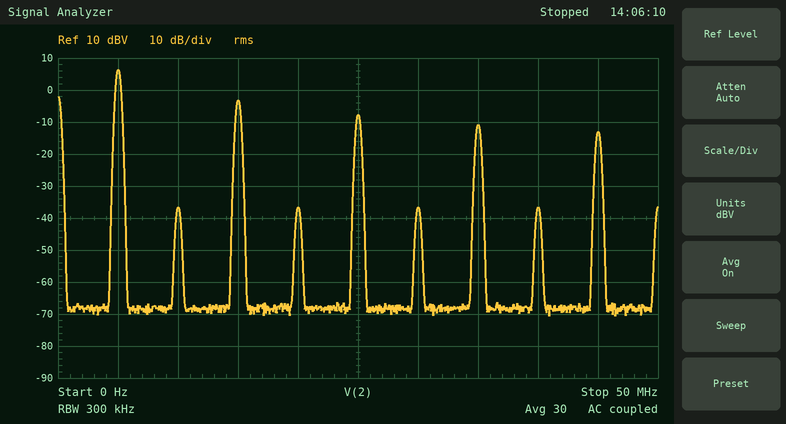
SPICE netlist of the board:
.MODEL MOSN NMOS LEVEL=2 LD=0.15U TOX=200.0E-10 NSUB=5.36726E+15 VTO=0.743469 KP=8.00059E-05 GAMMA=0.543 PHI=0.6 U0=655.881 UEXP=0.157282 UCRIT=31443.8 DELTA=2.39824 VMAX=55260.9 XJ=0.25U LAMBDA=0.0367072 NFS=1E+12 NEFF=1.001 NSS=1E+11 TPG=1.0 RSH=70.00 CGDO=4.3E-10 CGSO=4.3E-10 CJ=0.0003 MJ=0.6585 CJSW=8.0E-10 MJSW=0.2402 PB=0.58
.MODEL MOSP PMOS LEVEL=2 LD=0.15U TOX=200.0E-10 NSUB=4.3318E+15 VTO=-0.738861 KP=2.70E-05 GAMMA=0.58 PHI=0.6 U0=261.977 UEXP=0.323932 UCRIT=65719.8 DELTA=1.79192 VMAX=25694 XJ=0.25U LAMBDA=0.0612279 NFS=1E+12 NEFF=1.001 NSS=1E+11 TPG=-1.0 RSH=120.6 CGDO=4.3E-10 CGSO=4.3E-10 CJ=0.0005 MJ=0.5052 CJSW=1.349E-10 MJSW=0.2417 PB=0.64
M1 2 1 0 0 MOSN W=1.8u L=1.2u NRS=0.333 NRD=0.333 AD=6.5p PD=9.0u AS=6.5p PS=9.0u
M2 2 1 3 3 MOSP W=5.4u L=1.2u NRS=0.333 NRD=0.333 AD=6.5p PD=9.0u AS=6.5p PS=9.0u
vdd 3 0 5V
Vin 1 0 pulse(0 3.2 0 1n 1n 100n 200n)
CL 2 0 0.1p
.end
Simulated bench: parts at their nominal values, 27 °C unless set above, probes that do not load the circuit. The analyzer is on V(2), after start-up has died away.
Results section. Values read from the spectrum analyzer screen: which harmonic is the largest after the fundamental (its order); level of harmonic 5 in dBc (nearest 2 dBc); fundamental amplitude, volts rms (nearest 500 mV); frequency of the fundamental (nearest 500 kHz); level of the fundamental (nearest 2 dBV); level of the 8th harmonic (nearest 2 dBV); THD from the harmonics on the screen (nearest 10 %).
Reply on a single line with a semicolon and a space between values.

3; -14 dBc; 2.0 V; 5.0 MHz; 6 dBV; -36 dBV; 40 %
